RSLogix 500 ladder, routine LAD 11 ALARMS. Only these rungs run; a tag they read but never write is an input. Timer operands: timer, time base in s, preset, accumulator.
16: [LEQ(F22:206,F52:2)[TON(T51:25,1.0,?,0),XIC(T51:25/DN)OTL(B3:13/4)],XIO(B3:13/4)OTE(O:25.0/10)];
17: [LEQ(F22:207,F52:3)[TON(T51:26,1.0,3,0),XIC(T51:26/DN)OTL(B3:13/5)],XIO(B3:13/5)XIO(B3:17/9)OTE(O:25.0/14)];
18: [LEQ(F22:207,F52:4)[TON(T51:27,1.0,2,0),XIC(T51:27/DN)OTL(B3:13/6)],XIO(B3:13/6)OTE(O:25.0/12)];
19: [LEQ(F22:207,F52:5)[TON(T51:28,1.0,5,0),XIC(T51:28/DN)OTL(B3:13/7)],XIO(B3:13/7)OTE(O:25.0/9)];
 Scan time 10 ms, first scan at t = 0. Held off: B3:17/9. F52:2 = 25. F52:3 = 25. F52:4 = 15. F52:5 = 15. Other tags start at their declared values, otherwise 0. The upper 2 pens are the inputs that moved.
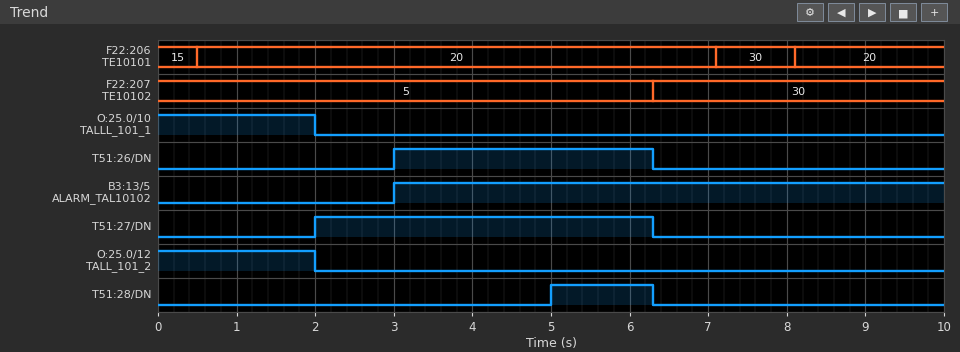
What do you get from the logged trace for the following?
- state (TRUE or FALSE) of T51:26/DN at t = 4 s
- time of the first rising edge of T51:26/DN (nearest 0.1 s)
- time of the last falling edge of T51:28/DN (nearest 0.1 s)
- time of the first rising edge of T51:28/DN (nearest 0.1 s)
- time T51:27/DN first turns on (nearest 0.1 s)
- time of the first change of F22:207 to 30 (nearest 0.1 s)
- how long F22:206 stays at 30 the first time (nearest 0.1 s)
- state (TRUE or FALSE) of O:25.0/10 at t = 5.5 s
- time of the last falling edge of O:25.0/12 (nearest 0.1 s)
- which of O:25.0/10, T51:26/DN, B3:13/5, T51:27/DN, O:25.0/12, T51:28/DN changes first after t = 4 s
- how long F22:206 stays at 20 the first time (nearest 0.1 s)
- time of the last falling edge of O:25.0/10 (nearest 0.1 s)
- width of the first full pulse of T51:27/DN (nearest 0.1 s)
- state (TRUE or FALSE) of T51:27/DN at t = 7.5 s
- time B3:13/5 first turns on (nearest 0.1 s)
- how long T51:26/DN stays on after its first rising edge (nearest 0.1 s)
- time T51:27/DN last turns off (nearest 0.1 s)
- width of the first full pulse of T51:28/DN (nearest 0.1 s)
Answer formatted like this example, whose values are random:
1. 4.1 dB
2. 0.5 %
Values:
1. TRUE
2. 3.0 s
3. 6.3 s
4. 5.0 s
5. 2.0 s
6. 6.3 s
7. 1.0 s
8. FALSE
9. 2.0 s
10. T51:28/DN
11. 6.6 s
12. 2.0 s
13. 4.3 s
14. FALSE
15. 3.0 s
16. 3.3 s
17. 6.3 s
18. 1.3 s
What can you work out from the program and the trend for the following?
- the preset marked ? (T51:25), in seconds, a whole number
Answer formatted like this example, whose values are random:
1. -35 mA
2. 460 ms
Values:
1. 2 s
